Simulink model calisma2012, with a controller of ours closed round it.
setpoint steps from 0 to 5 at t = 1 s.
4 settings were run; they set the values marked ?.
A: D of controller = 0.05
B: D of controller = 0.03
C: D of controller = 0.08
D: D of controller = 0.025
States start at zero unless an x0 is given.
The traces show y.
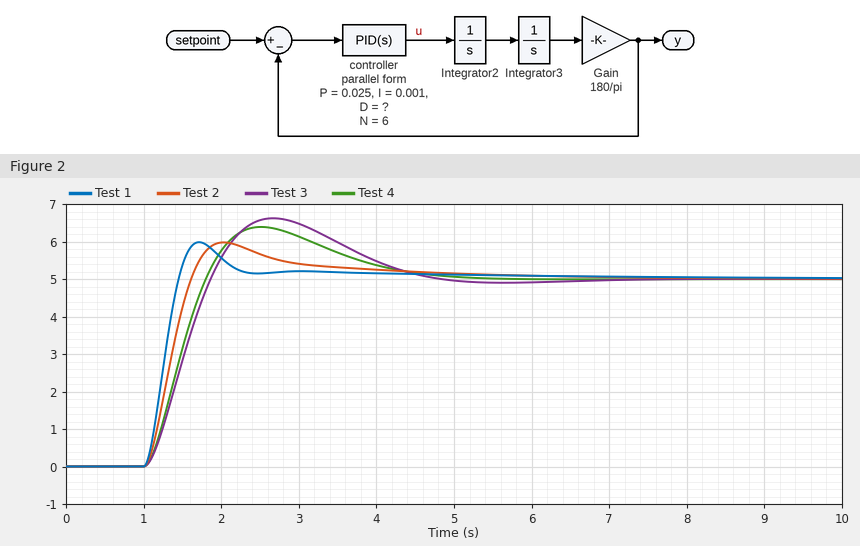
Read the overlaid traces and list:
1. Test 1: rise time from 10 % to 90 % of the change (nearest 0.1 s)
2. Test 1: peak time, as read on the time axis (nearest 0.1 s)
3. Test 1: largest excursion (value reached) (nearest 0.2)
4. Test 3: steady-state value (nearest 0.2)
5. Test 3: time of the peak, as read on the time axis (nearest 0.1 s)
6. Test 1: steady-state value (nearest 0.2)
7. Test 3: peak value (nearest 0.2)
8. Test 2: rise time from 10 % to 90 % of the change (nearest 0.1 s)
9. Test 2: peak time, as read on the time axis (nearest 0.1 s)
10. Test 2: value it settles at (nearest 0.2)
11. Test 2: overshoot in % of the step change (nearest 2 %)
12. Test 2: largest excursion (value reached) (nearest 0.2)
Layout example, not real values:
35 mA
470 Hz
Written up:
0.3 s
1.7 s
6.0
5.0
2.7 s
5.0
6.6
0.4 s
2.0 s
5.0
20 %
6.0
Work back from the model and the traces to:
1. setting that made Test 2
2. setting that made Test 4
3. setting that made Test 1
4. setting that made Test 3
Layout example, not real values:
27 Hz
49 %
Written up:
A
B
C
D
